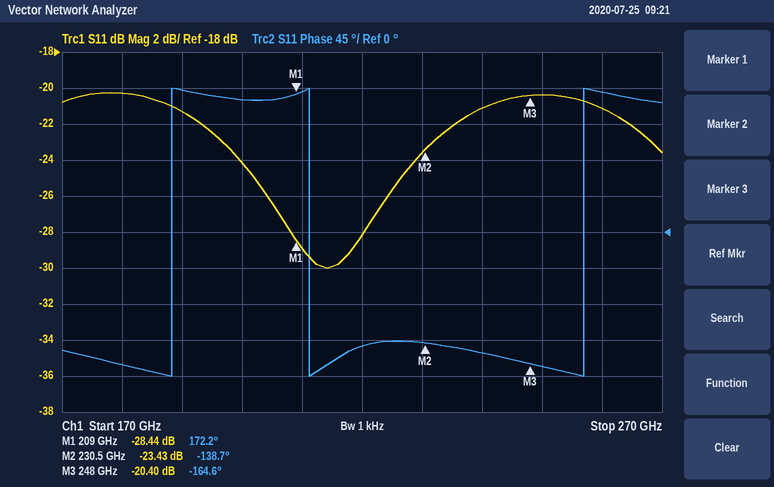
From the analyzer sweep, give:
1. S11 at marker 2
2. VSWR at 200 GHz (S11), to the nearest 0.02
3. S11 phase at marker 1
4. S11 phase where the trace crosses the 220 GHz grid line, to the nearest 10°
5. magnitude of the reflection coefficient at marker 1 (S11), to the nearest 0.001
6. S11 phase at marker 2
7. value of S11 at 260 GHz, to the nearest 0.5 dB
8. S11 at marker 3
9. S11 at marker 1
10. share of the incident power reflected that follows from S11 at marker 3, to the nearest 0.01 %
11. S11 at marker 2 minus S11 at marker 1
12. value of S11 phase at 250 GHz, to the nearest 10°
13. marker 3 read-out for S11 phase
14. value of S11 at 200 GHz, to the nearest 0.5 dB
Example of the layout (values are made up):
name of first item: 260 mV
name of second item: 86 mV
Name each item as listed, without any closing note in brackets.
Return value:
S11 at marker 2: -23.43 dB
VSWR at 200 GHz (S11), to the nearest 0.02: 1.14
S11 phase at marker 1: 172.2°
S11 phase where the trace crosses the 220 GHz grid line, to the nearest 10°: -140°
magnitude of the reflection coefficient at marker 1 (S11), to the nearest 0.001: 0.038
S11 phase at marker 2: -138.7°
value of S11 at 260 GHz, to the nearest 0.5 dB: -21.0 dB
S11 at marker 3: -20.40 dB
S11 at marker 1: -28.44 dB
share of the incident power reflected that follows from S11 at marker 3, to the nearest 0.01 %: 0.91 %
S11 at marker 2 minus S11 at marker 1: 5.01 dB
value of S11 phase at 250 GHz, to the nearest 10°: -170°
marker 3 read-out for S11 phase: -164.6°
value of S11 at 200 GHz, to the nearest 0.5 dB: -24.0 dB
